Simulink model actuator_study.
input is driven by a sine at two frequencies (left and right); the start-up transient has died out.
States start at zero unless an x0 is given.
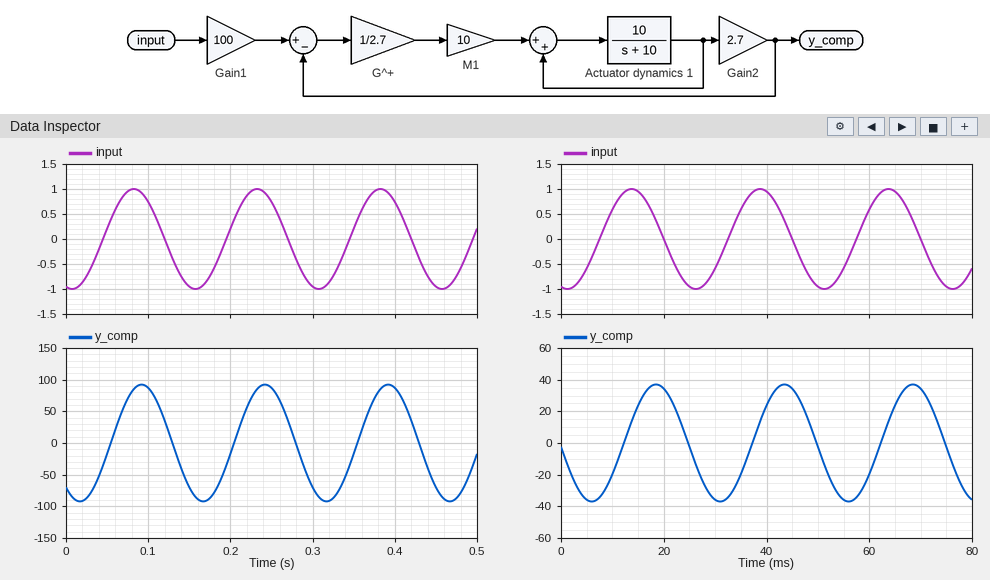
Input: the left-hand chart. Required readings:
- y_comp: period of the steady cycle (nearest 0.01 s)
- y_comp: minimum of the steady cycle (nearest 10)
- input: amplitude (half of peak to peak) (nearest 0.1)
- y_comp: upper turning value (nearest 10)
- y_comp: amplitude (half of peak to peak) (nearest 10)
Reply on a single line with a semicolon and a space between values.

0.15 s; -90; 1.0; 90; 90
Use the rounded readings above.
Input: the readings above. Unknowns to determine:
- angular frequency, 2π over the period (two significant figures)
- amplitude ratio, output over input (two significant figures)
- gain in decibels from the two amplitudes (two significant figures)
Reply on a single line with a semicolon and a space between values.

42 rad/s; 90; 39 dB
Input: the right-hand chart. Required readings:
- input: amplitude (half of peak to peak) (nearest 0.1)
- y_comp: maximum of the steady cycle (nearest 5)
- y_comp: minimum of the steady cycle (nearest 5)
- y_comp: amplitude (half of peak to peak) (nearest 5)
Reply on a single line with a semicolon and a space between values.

1.0; 35; -35; 35
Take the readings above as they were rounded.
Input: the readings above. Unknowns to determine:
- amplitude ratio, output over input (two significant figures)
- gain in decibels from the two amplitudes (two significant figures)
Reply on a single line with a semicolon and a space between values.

35; 31 dB
